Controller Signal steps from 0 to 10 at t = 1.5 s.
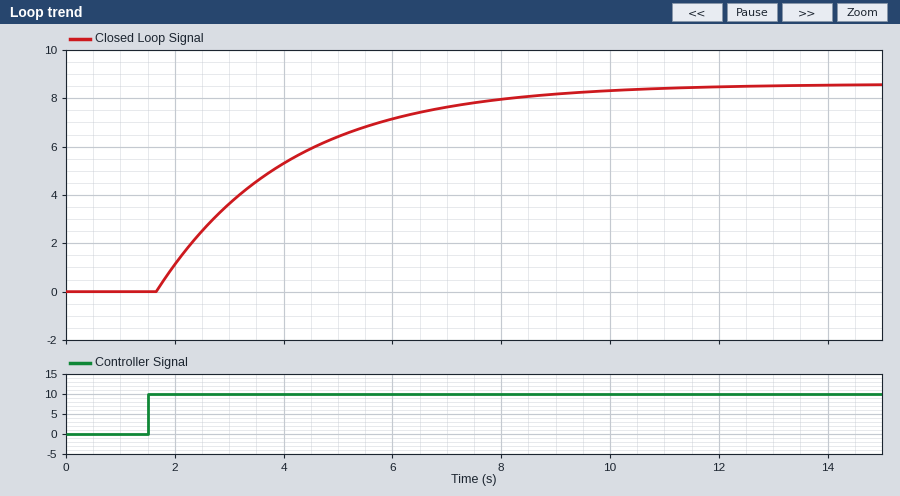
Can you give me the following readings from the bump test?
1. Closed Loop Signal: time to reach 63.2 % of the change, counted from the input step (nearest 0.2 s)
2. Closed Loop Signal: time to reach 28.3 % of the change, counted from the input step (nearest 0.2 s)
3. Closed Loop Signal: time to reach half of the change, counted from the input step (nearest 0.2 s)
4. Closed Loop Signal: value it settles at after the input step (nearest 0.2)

2.6 s
1.0 s
1.8 s
8.6
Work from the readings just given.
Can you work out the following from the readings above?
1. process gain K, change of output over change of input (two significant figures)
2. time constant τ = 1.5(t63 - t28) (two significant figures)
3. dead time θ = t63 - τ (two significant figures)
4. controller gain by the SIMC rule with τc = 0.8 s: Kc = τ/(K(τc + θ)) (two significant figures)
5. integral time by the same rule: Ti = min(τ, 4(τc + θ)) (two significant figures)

0.86
2.4 s
0.20 s
2.8
2.4 s
